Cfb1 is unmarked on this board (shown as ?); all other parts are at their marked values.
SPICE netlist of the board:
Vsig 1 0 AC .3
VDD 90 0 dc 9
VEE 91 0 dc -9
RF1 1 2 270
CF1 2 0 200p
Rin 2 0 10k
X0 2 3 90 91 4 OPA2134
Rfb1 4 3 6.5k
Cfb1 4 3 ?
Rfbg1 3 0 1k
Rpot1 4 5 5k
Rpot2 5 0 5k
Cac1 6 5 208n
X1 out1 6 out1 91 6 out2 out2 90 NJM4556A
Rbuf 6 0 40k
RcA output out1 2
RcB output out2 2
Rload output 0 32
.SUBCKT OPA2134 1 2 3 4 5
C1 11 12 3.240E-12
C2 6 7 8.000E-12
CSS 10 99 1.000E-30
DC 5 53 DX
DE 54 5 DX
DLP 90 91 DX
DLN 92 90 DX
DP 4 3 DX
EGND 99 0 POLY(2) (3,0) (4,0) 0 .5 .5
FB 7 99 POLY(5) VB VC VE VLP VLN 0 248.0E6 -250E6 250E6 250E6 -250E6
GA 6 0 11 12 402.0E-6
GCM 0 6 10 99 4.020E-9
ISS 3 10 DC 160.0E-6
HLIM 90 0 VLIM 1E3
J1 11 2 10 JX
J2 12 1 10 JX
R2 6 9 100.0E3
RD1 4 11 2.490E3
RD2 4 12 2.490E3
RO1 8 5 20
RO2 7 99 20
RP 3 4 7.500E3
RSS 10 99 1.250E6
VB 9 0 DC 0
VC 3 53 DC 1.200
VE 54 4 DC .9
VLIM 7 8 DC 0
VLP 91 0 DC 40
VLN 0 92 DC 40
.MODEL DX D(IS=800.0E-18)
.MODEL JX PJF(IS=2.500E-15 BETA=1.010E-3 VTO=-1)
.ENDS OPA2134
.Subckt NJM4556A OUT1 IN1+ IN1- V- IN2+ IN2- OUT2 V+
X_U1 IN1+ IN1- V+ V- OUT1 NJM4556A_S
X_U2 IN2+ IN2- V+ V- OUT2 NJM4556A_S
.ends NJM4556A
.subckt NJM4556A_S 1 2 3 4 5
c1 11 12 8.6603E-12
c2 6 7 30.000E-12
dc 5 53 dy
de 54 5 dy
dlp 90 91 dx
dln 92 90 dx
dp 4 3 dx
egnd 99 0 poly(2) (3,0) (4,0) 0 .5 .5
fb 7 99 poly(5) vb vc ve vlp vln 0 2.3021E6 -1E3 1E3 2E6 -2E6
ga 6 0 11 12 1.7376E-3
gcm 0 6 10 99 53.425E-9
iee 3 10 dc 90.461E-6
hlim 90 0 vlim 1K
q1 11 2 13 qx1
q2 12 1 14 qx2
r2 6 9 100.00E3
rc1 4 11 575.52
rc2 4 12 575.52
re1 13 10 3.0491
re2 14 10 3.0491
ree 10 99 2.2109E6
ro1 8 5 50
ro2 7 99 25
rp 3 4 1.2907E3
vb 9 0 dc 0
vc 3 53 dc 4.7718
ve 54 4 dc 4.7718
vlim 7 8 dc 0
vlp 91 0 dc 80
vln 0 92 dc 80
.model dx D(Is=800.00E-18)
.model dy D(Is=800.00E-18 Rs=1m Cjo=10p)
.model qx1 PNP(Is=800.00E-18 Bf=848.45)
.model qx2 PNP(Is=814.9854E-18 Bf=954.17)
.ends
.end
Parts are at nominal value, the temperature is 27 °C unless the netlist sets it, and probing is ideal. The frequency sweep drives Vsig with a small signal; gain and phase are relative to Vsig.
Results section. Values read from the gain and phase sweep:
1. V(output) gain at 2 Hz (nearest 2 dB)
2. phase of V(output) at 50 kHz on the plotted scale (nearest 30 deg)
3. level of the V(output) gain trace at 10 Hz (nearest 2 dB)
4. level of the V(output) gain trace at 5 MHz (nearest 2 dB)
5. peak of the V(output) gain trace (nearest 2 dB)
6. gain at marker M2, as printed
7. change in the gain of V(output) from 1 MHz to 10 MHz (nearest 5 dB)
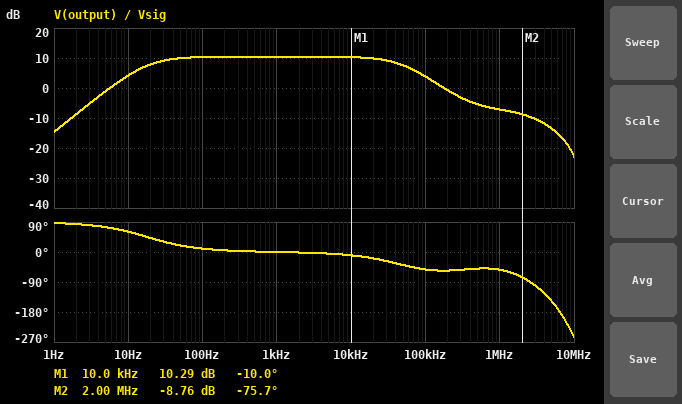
-8 dB
-30 deg
4 dB
-14 dB
10 dB
-8.76 dB
-15 dB
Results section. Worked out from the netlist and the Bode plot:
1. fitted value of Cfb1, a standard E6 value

470 pF
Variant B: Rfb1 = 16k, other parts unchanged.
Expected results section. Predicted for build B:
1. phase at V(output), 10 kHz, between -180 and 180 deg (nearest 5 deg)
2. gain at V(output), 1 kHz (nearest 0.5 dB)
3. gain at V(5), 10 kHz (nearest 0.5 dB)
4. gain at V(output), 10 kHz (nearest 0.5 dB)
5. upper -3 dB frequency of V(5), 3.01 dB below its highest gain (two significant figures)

-25 deg
17.5 dB
17.0 dB
16.5 dB
18 kHz
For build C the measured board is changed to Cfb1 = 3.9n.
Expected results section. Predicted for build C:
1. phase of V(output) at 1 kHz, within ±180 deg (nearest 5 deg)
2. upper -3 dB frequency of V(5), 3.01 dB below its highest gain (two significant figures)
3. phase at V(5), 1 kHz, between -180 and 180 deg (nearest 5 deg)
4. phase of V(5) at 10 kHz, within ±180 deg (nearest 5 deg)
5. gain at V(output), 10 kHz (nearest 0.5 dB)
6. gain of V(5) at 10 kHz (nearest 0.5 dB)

-5 deg
5.6 kHz
-10 deg
-45 deg
5.0 dB
5.5 dB
